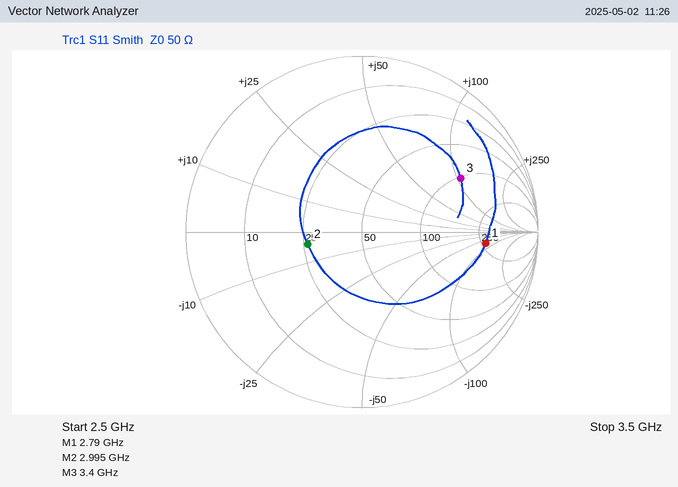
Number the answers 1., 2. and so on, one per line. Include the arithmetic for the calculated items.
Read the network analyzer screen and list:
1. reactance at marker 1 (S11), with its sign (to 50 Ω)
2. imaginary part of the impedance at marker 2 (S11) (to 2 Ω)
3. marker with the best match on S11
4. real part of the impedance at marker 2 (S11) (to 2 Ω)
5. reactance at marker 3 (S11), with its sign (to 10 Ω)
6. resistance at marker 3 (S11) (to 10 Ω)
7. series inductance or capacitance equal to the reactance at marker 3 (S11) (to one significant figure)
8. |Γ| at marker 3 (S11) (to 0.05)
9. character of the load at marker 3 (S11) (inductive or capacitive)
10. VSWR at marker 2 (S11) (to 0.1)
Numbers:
1. -50 Ω
2. -4 Ω
3. marker 2
4. 26 Ω
5. +110 Ω
6. 100 Ω
7. L = 110 Ω/(2π × 3.4 GHz) ≈ 5 nH
8. 0.65
9. inductive
10. 1.9
